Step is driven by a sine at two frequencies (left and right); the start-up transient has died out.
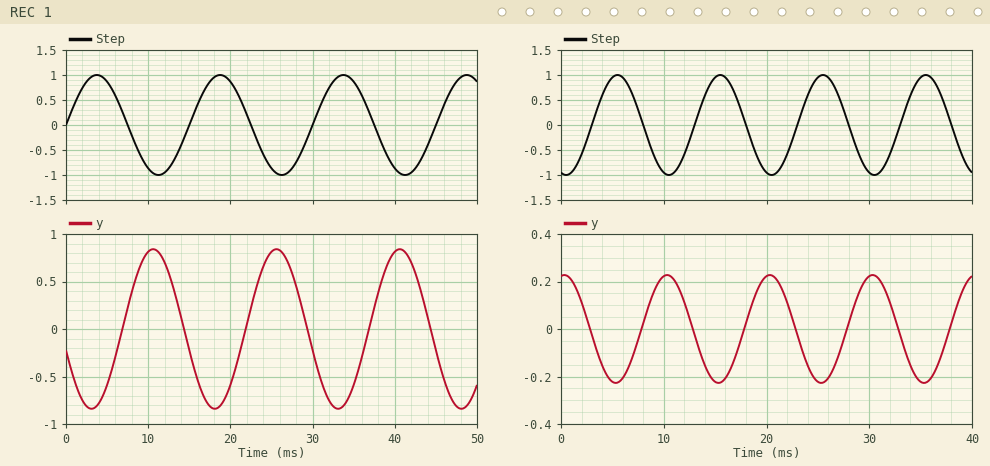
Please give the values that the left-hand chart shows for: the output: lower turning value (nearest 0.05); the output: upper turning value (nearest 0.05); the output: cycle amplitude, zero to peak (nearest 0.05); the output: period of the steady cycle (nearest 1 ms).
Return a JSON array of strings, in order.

["-0.85", "0.85", "0.85", "15 ms"]
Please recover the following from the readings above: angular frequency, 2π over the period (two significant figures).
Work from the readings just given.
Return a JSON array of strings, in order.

["0.42 rad/ms"]
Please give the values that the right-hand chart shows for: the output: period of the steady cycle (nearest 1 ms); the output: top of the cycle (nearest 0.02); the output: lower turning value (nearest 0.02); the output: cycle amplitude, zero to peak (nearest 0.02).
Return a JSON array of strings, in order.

["10 ms", "0.22", "-0.22", "0.22"]
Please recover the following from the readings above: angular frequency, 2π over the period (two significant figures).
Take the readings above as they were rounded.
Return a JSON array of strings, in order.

["0.63 rad/ms"]
